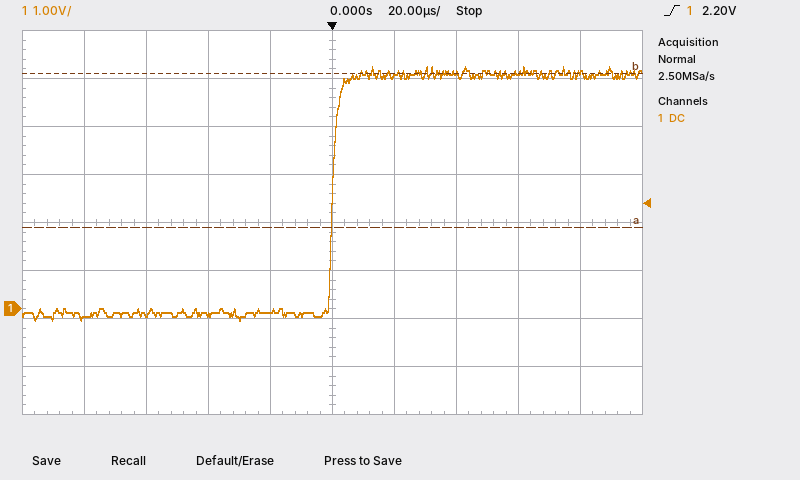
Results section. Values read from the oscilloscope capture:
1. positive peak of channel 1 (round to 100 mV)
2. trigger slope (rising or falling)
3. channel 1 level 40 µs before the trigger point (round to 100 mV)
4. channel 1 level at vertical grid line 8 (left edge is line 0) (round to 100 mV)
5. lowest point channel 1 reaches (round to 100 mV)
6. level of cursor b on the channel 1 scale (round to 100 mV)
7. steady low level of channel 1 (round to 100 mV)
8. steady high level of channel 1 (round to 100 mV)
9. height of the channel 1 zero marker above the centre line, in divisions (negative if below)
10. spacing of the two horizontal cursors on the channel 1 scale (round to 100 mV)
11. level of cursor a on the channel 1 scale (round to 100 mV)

5.0 V
rising
-100 mV
4.9 V
-200 mV
4.9 V
-100 mV
4.9 V
-1.8 div
3.2 V
1.7 V
